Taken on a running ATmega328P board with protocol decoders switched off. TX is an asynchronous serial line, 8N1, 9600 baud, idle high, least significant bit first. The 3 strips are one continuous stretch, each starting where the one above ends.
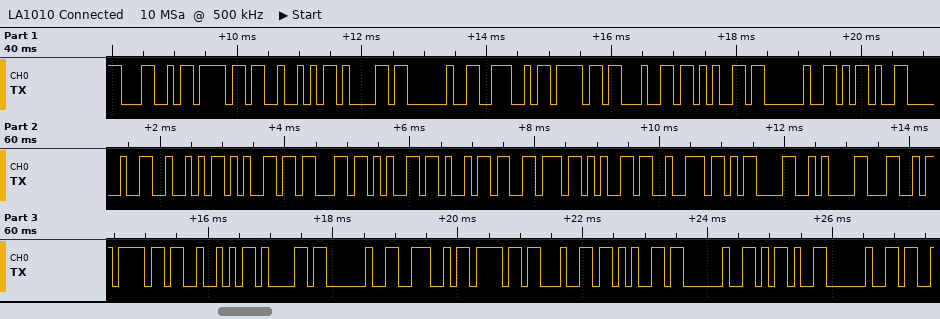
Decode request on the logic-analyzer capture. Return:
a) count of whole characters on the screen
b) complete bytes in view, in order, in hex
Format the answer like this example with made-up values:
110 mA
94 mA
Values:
34
4C 6F 52 61 20 4E 6F 64 65 20 2D 20 52 65 63 65 69 76 65 72 0D 0A 4C 6F 52 61 20 4E 6F 64 65 20 2D 20
